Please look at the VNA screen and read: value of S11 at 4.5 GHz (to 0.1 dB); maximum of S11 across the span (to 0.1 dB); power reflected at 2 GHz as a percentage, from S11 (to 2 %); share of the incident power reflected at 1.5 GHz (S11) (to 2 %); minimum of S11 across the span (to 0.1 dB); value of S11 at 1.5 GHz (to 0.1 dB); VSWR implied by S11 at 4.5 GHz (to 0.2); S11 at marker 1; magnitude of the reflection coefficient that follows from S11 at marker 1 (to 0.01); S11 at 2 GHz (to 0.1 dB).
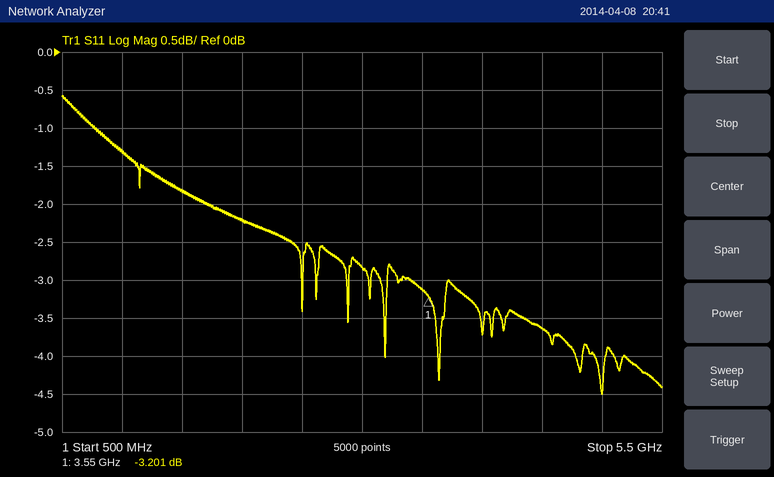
-3.6 dB
-0.6 dB
60 %
66 %
-4.5 dB
-1.8 dB
4.8
-3.201 dB
0.69
-2.2 dB
